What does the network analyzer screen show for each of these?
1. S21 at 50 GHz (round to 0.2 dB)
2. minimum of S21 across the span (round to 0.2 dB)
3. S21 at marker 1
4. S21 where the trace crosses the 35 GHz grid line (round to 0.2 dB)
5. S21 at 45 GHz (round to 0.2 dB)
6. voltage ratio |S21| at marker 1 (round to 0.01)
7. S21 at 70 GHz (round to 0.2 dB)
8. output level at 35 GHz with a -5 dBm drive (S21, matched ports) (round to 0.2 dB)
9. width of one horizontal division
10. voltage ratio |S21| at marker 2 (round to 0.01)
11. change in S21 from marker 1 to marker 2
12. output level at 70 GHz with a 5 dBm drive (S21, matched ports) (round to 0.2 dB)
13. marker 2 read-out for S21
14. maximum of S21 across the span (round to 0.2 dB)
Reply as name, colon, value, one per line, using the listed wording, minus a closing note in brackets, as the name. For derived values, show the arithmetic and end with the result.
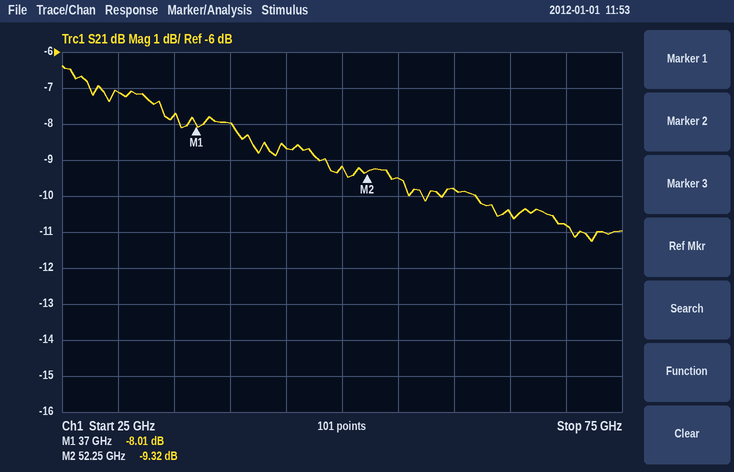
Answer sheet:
S21 at 50 GHz: -9.2 dB
minimum of S21 across the span: -11.2 dB
S21 at marker 1: -8.01 dB
S21 where the trace crosses the 35 GHz grid line: -7.8 dB
S21 at 45 GHz: -8.6 dB
voltage ratio |S21| at marker 1: 10^(-8.01/20) ≈ 0.40
S21 at 70 GHz: -10.8 dB
output level at 35 GHz with a -5 dBm drive (S21, matched ports): -5 dBm + (-7.8 dB) = -12.8 dBm
width of one horizontal division: 5 GHz
voltage ratio |S21| at marker 2: 10^(-9.32/20) ≈ 0.34
change in S21 from marker 1 to marker 2: -9.32 − (-8.01) = -1.31 dB
output level at 70 GHz with a 5 dBm drive (S21, matched ports): 5 dBm + (-10.8 dB) = -5.8 dBm
marker 2 read-out for S21: -9.32 dB
maximum of S21 across the span: -6.4 dB
